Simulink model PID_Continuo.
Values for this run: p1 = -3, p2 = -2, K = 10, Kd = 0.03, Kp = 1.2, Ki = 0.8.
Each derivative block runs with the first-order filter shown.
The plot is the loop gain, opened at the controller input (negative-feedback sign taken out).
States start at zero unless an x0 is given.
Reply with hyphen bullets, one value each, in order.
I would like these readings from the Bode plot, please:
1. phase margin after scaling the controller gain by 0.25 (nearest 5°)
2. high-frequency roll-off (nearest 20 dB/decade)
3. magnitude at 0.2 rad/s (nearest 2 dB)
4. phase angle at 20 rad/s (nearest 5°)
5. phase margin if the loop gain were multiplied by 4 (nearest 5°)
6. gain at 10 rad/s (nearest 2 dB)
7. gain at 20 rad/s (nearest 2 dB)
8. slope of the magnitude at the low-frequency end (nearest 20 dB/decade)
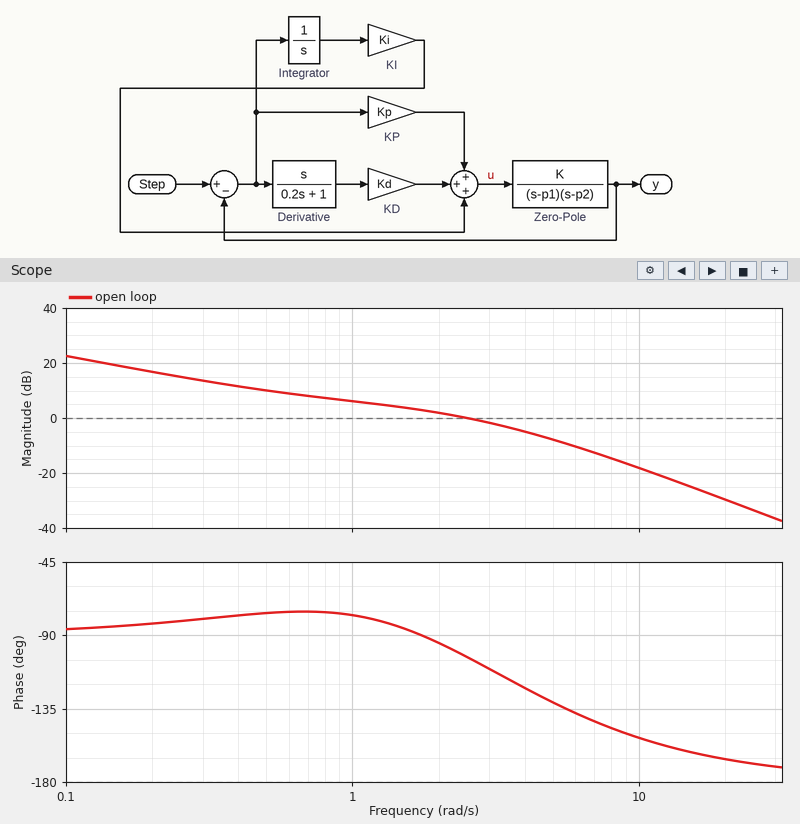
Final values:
- 100°
- -40 dB/decade
- 16 dB
- -165°
- 40°
- -18 dB
- -30 dB
- -20 dB/decade
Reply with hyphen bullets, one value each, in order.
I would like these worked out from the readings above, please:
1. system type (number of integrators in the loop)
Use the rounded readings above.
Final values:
- 1
